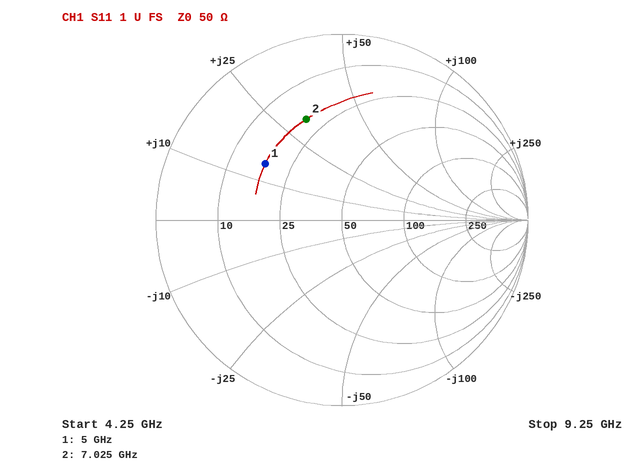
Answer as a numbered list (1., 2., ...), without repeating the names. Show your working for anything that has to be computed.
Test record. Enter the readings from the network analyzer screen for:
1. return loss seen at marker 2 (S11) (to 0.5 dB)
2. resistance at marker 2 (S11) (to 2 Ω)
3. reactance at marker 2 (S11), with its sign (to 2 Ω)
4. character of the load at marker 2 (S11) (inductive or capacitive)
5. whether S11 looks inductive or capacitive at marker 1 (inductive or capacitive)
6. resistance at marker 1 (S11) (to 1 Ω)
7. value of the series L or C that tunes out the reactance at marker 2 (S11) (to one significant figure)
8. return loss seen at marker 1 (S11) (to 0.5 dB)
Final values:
1. 5.0 dB
2. 20 Ω
3. +32 Ω
4. inductive
5. inductive
6. 18 Ω
7. C = 1/(2π × 7.025 GHz × 32 Ω) ≈ 708 fF, so 700 fF to one significant figure
8. 6.0 dB
